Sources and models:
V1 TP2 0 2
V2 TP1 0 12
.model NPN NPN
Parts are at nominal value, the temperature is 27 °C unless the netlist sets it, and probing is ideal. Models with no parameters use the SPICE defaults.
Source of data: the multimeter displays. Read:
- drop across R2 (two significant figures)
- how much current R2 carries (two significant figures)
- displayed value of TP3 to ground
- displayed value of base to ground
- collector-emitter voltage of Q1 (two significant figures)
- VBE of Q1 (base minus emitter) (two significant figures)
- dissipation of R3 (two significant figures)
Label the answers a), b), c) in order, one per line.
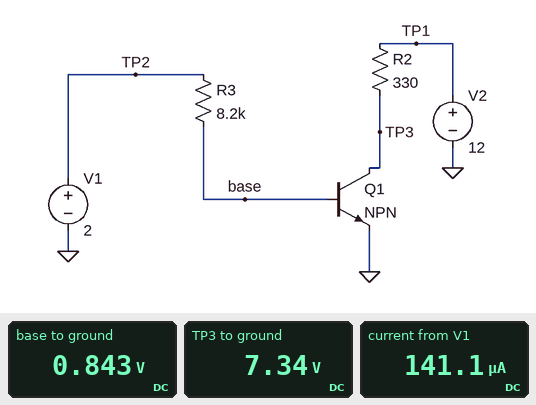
a) 4.7 V
b) 14 mA
c) 7.34 V
d) 0.843 V
e) 7.3 V
f) 840 mV
g) 160 µW
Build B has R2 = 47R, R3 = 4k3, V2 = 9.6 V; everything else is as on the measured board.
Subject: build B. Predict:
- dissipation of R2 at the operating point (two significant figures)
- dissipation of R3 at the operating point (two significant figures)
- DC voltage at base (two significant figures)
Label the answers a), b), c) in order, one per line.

a) 33 mW
b) 300 µW
c) 860 mV
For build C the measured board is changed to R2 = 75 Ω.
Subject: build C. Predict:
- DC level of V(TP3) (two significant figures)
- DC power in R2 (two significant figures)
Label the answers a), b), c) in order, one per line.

a) 11 V
b) 15 mW
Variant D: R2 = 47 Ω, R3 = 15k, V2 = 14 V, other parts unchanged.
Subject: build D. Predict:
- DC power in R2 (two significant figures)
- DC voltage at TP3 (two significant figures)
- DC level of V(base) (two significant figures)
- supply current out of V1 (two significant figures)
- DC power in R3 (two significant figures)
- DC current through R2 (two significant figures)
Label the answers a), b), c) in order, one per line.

a) 2.9 mW
b) 14 V
c) 830 mV
d) 78 µA
e) 92 µW
f) 7.8 mA
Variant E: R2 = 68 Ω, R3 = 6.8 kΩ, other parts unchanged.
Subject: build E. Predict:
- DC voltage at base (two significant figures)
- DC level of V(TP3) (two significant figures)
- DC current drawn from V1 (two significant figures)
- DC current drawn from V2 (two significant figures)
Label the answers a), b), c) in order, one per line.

a) 850 mV
b) 11 V
c) 170 µA
d) 17 mA
